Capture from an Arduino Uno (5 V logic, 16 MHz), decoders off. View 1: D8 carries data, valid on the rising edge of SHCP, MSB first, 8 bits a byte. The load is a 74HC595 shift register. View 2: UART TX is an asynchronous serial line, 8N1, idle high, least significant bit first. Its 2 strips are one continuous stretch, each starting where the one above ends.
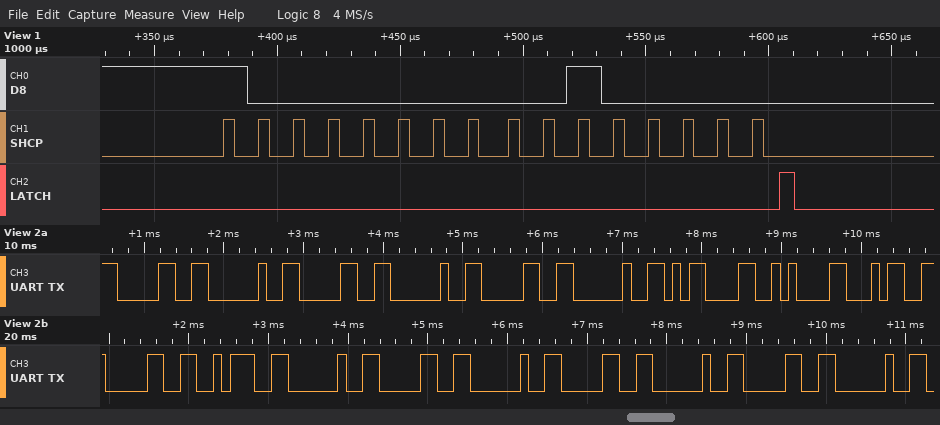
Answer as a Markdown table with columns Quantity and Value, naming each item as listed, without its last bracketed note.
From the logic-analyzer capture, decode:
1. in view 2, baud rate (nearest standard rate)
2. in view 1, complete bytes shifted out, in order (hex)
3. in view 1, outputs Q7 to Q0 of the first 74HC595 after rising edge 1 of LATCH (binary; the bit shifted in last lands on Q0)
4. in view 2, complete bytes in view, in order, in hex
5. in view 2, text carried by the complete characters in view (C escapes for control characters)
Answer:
| Quantity | Value |
|---|---|
| in view 2, baud rate | 9600 baud |
| in view 1, complete bytes shifted out, in order | 0x80 0x20 |
| in view 1, outputs Q7 to Q0 of the first 74HC595 after rising edge 1 of LATCH | 00100000 |
| in view 2, complete bytes in view, in order, in hex | 30 20 30 20 30 20 0D 0A 34 30 3A 20 30 20 30 20 30 20 |
| in view 2, text carried by the complete characters in view | "0 0 0 \r\n40: 0 0 0 " |
